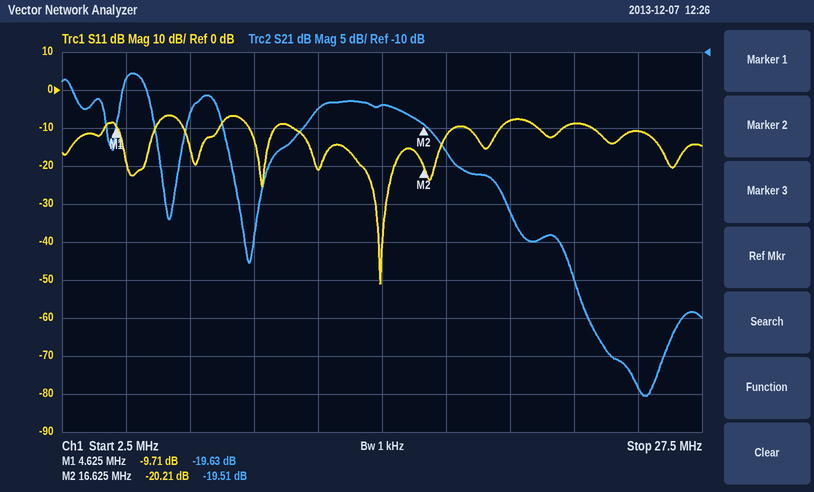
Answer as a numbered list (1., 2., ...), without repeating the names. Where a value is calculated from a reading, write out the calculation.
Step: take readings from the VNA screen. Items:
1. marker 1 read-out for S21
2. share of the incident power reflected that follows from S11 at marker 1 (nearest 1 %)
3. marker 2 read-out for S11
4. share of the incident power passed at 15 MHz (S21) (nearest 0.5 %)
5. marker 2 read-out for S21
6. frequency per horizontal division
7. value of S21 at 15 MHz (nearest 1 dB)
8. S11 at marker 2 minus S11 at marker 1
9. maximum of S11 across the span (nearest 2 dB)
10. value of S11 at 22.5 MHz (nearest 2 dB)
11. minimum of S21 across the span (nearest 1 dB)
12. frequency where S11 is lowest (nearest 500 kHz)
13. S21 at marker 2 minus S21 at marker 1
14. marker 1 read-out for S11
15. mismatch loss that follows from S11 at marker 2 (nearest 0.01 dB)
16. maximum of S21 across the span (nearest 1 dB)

1. -19.63 dB
2. 10^(-9.71/10) ≈ 11 %
3. -20.21 dB
4. 10^(-17/10) ≈ 2.0 %
5. -19.51 dB
6. 2.5 MHz
7. -17 dB
8. -20.21 − (-9.71) = -10.50 dB
9. -6 dB
10. -8 dB
11. -55 dB
12. 15.0 MHz
13. -19.51 − (-19.63) = 0.12 dB
14. -9.71 dB
15. −10 log10(1 − 10^(-20.21/10)) ≈ 0.04 dB
16. -13 dB
